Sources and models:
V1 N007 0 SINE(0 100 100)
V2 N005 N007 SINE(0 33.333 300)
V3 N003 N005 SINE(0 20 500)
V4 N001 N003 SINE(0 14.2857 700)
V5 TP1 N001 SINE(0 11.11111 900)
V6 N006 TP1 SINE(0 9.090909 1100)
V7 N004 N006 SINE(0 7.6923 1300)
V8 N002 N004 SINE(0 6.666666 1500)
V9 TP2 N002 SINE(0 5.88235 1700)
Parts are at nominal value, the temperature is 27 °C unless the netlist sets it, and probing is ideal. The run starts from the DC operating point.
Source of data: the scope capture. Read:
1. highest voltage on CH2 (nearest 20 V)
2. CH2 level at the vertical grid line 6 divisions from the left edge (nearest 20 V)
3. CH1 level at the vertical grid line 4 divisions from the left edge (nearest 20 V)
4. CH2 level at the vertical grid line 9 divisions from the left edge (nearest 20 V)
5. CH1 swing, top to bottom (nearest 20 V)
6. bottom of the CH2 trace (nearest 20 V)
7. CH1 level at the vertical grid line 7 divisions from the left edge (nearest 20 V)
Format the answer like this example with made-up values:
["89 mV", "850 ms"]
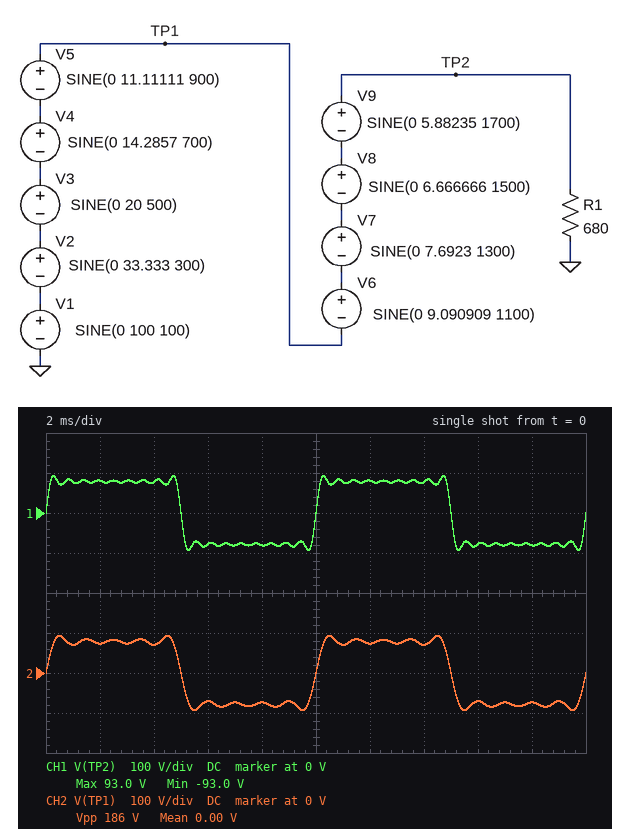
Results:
["100 V", "80 V", "-80 V", "-80 V", "180 V", "-100 V", "80 V"]
